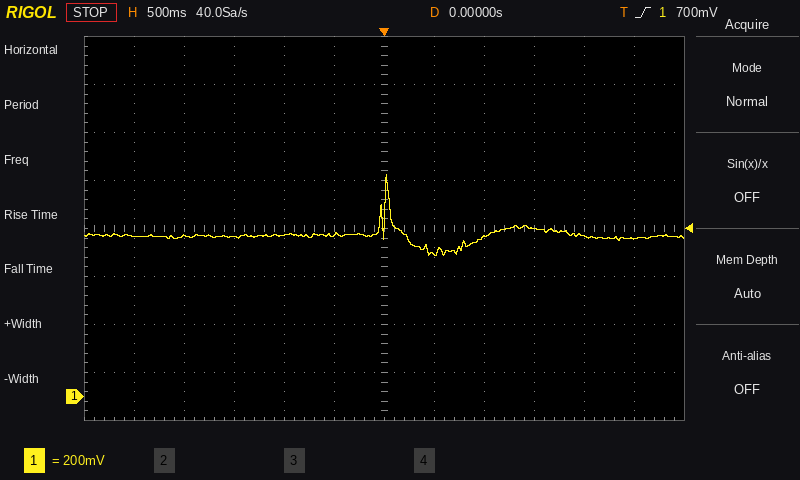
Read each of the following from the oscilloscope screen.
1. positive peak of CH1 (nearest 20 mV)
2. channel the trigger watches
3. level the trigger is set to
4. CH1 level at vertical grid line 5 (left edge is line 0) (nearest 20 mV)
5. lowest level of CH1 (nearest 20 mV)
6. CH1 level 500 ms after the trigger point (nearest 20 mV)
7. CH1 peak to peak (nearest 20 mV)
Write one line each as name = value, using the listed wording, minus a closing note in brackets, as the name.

positive peak of CH1 = 920 mV
channel the trigger watches = CH1
level the trigger is set to = 700 mV
CH1 level at vertical grid line 5 (left edge is line 0) = 680 mV
lowest level of CH1 = 580 mV
CH1 level 500 ms after the trigger point = 600 mV
CH1 peak to peak = 340 mV
